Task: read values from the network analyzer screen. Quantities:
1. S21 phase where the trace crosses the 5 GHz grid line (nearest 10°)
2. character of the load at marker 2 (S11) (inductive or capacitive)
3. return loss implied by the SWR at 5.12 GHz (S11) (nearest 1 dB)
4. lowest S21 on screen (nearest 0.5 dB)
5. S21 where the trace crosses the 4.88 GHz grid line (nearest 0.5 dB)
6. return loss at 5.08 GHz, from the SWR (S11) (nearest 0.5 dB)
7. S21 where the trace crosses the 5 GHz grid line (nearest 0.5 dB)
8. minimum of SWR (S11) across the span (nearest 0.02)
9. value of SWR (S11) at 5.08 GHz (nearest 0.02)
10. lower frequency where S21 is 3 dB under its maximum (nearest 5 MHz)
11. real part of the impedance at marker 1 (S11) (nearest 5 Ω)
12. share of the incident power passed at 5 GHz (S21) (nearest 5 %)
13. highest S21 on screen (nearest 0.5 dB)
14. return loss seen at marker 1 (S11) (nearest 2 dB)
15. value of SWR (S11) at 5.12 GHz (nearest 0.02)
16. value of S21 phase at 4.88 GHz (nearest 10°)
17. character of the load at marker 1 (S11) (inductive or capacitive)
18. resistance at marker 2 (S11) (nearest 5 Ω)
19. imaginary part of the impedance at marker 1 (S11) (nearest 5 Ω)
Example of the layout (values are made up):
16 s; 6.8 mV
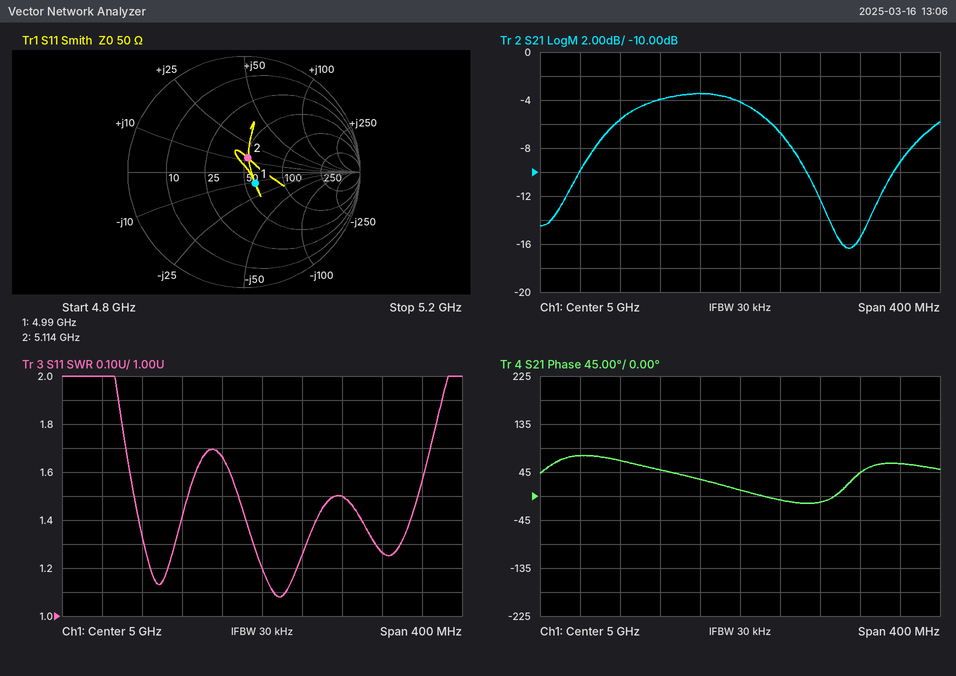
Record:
10°; inductive; 19 dB; -16.5 dB; -5.5 dB; 14.0 dB; -4.0 dB; 1.08; 1.50; 4.870 GHz; 60 Ω; 40 %; -3.5 dB; 18 dB; 1.26; 70°; capacitive; 50 Ω; -10 Ω
